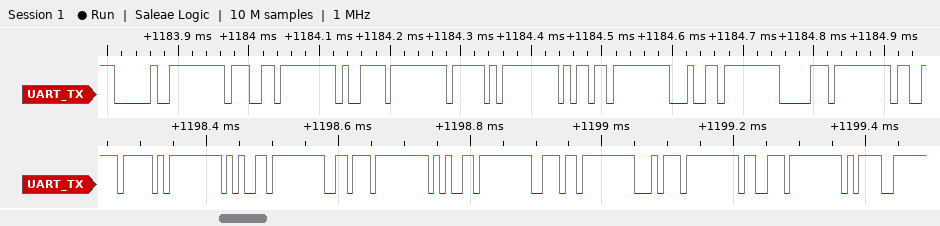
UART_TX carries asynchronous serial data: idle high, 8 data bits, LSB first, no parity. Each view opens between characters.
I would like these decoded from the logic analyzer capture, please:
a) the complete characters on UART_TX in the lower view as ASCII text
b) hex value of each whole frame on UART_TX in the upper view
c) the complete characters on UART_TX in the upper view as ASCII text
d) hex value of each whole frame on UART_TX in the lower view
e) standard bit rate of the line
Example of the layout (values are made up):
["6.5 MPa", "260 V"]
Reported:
["\"_events=\"", "20, 67, 79, 5F, 6D, 64, 70", "\" gy_mdp\"", "5F, 65, 76, 65, 6E, 74, 73, 3D", "115200 baud"]
